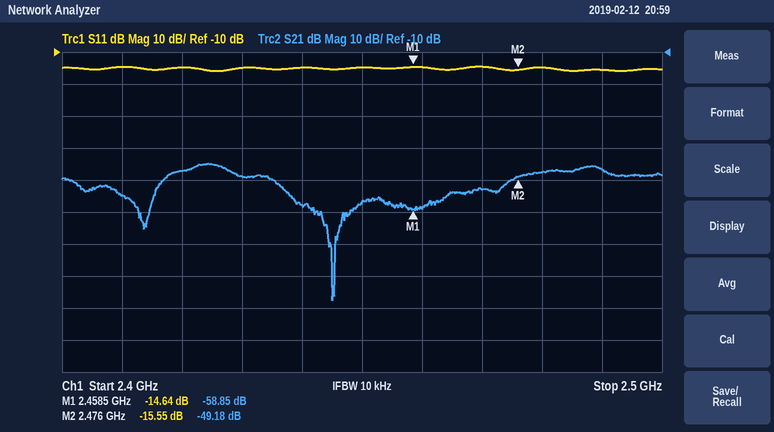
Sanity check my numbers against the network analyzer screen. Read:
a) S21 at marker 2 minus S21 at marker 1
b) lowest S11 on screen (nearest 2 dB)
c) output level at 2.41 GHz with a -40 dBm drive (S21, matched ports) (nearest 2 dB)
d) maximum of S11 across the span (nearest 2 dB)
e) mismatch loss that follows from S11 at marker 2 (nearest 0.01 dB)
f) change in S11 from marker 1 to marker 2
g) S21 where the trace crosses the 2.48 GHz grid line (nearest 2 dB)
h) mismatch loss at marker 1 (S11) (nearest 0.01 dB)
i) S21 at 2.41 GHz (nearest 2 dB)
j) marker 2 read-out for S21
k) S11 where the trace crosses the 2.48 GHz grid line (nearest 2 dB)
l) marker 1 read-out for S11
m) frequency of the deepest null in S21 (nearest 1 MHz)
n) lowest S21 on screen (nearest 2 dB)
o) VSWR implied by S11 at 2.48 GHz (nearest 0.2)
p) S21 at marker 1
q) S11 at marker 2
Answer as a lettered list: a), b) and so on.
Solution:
a) 9.67 dB
b) -16 dB
c) -94 dBm
d) -14 dB
e) 0.12 dB
f) -0.91 dB
g) -48 dB
h) 0.15 dB
i) -54 dB
j) -49.18 dB
k) -14 dB
l) -14.64 dB
m) 2.445 GHz
n) -88 dB
o) 1.4
p) -58.85 dB
q) -15.55 dB
